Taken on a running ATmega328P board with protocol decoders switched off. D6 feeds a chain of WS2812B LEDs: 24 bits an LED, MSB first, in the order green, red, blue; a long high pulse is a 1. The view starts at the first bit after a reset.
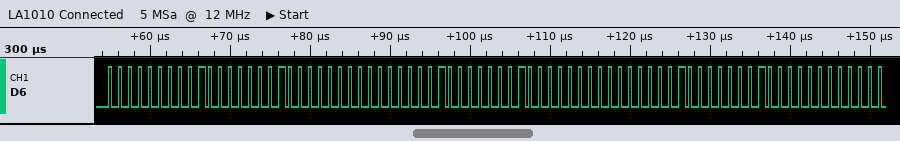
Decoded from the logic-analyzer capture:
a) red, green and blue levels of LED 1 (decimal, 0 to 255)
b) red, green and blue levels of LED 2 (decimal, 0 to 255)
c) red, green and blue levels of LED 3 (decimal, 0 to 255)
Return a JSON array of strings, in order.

["64, 0, 64", "64, 0, 64", "64, 0, 64"]
